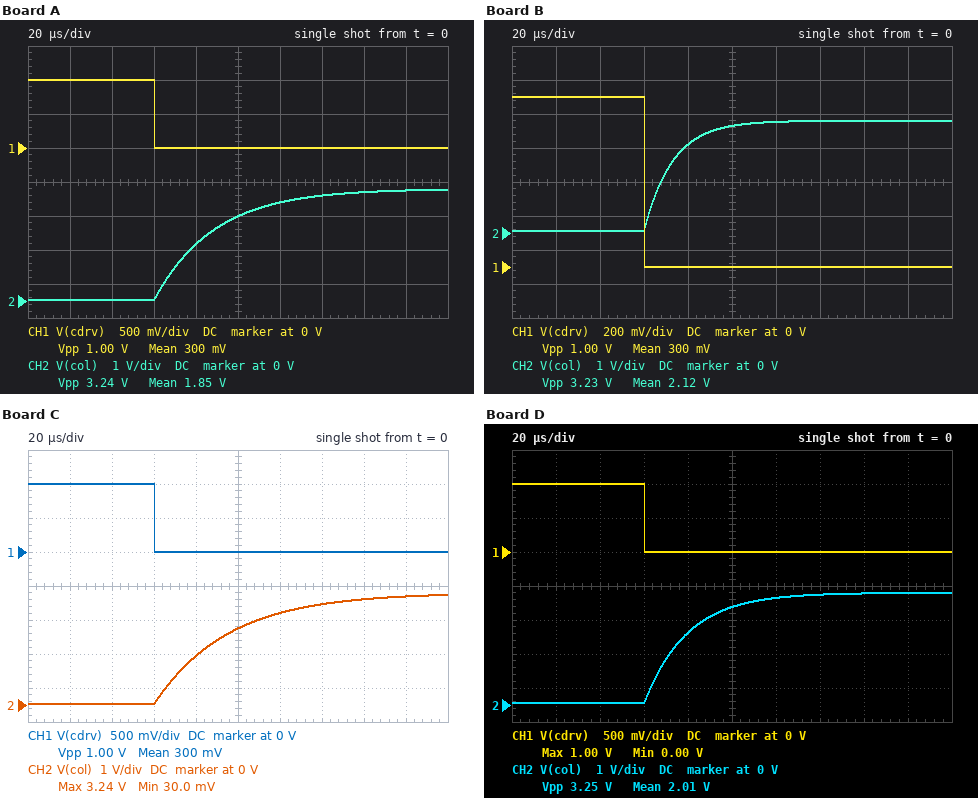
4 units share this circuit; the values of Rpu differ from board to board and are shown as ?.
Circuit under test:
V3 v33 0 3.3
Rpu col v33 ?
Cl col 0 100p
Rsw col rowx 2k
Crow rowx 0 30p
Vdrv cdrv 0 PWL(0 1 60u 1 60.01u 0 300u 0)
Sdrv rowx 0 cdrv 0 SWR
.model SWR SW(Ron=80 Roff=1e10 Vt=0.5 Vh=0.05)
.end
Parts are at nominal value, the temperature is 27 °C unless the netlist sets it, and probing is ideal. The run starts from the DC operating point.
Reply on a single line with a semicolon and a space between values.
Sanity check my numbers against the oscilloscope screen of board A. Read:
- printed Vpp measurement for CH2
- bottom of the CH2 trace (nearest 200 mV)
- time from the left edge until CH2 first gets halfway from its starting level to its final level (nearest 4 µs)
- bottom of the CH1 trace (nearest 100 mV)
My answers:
3.24 V; 0 V; 80 µs; 0 V
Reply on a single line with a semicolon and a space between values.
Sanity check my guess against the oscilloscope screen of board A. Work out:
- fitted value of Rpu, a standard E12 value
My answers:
220 kΩ
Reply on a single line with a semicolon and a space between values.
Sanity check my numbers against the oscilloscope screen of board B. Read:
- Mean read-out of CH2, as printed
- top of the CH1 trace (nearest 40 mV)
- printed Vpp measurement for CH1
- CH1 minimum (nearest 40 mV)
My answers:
2.12 V; 1.00 V; 1.00 V; 0 V
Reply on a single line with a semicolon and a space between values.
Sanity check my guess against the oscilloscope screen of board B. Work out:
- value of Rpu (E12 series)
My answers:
100 kΩ
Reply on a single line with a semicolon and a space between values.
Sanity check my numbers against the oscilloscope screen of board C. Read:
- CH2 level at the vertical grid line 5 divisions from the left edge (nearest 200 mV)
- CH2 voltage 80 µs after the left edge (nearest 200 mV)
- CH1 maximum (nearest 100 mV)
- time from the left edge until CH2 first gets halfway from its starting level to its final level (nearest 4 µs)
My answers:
2.2 V; 1.4 V; 1.0 V; 84 µs
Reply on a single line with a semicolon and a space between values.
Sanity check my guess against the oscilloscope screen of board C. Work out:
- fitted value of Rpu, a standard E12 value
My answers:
270 kΩ
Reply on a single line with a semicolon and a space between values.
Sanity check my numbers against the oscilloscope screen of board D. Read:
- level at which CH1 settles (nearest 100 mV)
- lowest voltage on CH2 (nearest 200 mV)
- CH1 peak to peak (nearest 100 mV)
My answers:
0 V; 0 V; 1.0 V
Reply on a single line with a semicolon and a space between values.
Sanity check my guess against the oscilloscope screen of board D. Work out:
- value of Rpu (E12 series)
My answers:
150 kΩ
